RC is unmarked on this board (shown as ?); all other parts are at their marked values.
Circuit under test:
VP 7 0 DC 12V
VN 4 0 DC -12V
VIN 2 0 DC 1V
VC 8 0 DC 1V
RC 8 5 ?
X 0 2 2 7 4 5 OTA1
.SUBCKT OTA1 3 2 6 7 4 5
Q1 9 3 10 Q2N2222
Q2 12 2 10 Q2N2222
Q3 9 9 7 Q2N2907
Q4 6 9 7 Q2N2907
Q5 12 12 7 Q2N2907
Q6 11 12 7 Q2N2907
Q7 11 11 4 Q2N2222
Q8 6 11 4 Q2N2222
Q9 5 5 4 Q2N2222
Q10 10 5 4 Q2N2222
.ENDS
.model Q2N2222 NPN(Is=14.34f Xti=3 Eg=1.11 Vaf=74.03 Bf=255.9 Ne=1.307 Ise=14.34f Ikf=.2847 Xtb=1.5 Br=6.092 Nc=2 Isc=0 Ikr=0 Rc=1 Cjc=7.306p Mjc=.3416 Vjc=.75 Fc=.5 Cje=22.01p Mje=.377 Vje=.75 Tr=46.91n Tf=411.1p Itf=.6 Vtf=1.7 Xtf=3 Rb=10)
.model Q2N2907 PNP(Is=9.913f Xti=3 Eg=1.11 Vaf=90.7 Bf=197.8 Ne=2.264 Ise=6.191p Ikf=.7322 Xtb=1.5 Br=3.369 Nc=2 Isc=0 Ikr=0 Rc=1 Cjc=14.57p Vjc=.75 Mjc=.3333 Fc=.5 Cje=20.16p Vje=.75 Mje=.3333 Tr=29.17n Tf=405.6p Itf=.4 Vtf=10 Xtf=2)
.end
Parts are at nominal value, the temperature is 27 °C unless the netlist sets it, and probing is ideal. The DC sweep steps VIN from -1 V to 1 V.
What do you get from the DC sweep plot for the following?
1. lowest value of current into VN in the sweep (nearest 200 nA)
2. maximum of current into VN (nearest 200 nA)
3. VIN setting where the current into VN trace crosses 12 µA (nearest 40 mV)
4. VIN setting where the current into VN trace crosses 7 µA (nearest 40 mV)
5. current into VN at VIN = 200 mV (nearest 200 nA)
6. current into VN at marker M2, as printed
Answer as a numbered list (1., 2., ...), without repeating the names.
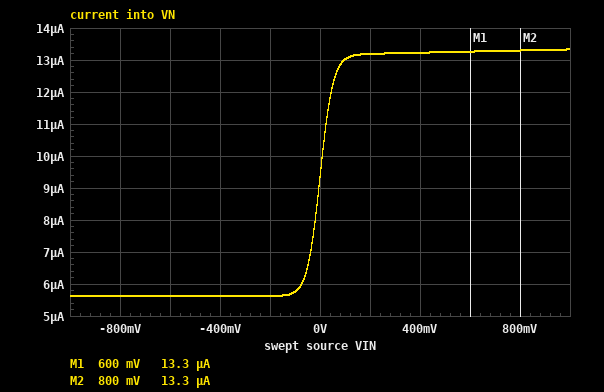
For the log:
1. 5.6 µA
2. 13.4 µA
3. 40 mV
4. -40 mV
5. 13.2 µA
6. 13.3 µA
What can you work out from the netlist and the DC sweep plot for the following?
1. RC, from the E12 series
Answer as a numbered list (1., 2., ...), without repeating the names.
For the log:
1. 4.7 MΩ
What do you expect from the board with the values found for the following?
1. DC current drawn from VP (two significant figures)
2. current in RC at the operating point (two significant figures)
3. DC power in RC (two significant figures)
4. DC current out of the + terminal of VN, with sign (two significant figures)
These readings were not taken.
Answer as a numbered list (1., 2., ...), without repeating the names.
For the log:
1. 6.6 µA
2. 2.7 µA
3. 33 µW
4. -13 µA
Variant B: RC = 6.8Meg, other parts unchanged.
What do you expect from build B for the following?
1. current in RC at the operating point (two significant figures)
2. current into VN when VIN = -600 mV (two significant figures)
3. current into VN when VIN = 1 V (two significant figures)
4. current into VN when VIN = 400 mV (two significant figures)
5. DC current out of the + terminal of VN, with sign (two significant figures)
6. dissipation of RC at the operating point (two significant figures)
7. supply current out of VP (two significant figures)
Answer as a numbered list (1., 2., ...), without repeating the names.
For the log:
1. 1.8 µA
2. 3.9 µA
3. 9.2 µA
4. 9.1 µA
5. -9.2 µA
6. 23 µW
7. 4.5 µA
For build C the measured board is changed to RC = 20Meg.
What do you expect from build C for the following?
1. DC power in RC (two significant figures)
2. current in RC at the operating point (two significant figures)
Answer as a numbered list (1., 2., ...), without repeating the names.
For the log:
1. 7.9 µW
2. 630 nA
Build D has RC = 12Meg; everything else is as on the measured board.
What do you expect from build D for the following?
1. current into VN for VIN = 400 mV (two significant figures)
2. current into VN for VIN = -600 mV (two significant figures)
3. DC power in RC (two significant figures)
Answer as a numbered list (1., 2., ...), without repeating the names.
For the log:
1. 5.1 µA
2. 2.2 µA
3. 13 µW
